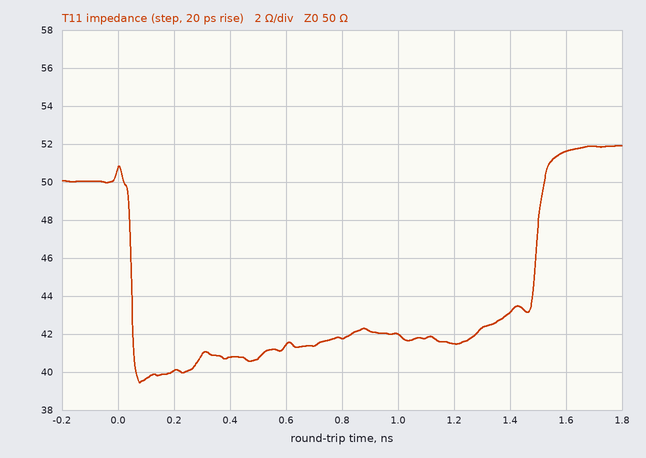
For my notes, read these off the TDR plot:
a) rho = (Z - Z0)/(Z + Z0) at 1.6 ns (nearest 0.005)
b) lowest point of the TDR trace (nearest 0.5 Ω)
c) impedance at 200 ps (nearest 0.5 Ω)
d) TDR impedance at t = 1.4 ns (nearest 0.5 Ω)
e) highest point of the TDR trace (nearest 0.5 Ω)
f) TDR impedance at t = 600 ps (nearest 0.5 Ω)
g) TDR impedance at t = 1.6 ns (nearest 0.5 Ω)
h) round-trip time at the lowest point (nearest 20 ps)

+0.015
39.5 Ω
40.0 Ω
43.0 Ω
52.0 Ω
41.5 Ω
51.5 Ω
80 ps
